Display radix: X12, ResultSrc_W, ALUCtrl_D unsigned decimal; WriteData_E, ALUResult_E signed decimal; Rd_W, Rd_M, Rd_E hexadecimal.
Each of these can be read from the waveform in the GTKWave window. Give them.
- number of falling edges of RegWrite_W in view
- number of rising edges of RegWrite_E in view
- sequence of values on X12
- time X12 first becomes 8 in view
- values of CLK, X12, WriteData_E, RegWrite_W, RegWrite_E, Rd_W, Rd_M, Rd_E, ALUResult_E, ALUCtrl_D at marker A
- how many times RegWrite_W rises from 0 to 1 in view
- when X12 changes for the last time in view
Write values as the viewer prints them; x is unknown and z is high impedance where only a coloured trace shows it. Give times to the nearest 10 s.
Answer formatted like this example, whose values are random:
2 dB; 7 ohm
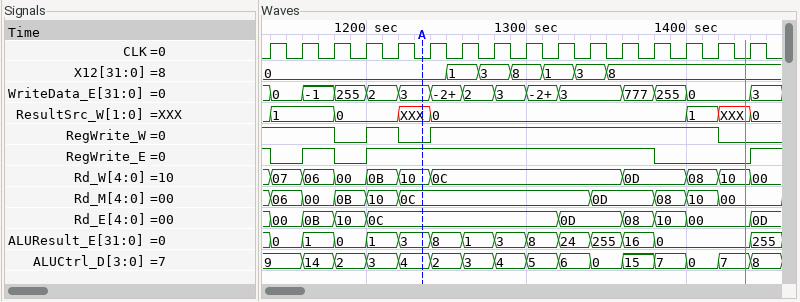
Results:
3; 3; 0, 1, 3, 8, 1, 3, 8; 1290 s; CLK=0, X12=0, WriteData_E=3, RegWrite_W=0, RegWrite_E=1, Rd_W=10, Rd_M=0C, Rd_E=0C, ALUResult_E=3, ALUCtrl_D=4; 2; 1350 s
